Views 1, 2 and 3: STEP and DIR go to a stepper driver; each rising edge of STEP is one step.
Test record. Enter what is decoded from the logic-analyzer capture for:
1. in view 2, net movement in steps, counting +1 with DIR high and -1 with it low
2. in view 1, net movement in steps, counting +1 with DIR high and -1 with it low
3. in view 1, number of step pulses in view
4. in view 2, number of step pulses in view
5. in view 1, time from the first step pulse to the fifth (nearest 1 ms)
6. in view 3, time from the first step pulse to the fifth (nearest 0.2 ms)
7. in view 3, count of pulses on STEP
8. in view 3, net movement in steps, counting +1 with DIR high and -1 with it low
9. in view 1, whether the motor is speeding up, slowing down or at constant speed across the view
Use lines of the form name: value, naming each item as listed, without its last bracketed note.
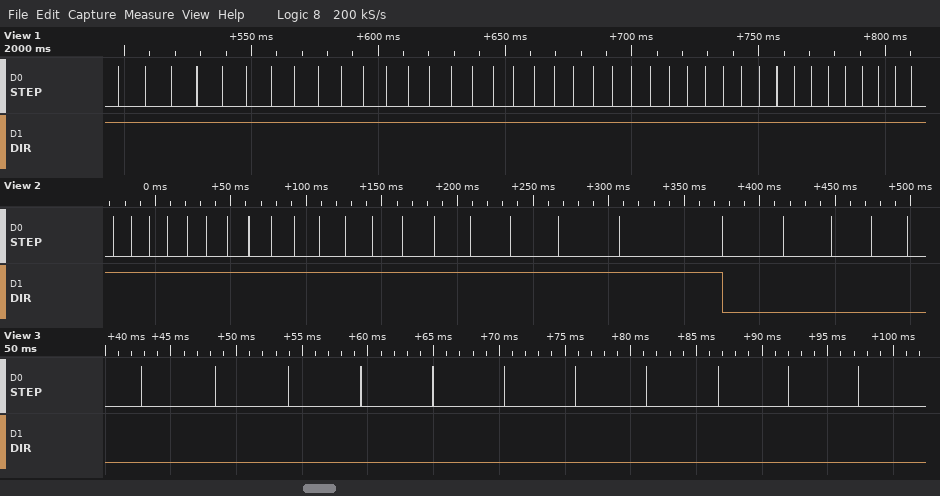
in view 2, net movement in steps, counting +1 with DIR high and -1 with it low: +14
in view 1, net movement in steps, counting +1 with DIR high and -1 with it low: +40
in view 1, number of step pulses in view: 40
in view 2, number of step pulses in view: 24
in view 1, time from the first step pulse to the fifth: 41 ms
in view 3, time from the first step pulse to the fifth: 22.2 ms
in view 3, count of pulses on STEP: 11
in view 3, net movement in steps, counting +1 with DIR high and -1 with it low: -11
in view 1, whether the motor is speeding up, slowing down or at constant speed across the view: speeding up
